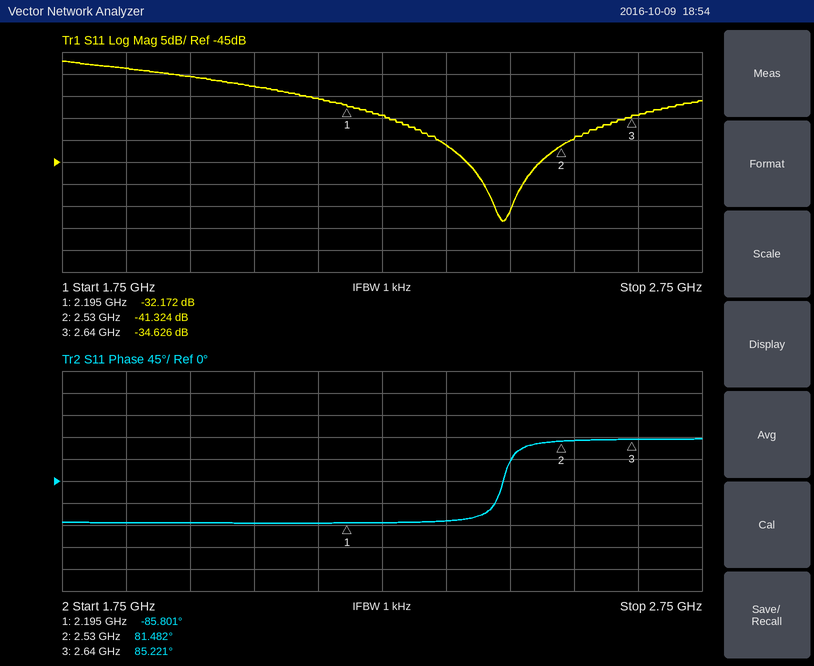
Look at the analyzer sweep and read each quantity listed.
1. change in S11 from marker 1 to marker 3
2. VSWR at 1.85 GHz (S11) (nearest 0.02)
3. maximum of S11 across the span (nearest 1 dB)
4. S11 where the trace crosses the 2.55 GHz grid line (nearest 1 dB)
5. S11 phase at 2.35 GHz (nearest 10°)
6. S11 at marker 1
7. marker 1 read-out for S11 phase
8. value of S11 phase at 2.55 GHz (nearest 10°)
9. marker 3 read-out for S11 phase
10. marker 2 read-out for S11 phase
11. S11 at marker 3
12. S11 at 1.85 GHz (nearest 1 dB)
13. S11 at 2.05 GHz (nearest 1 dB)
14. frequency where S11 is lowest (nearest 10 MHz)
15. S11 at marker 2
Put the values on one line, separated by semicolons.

-2.454 dB; 1.14; -22 dB; -40 dB; -80°; -32.172 dB; -85.801°; 80°; 85.221°; 81.482°; -34.626 dB; -24 dB; -28 dB; 2.44 GHz; -41.324 dB
